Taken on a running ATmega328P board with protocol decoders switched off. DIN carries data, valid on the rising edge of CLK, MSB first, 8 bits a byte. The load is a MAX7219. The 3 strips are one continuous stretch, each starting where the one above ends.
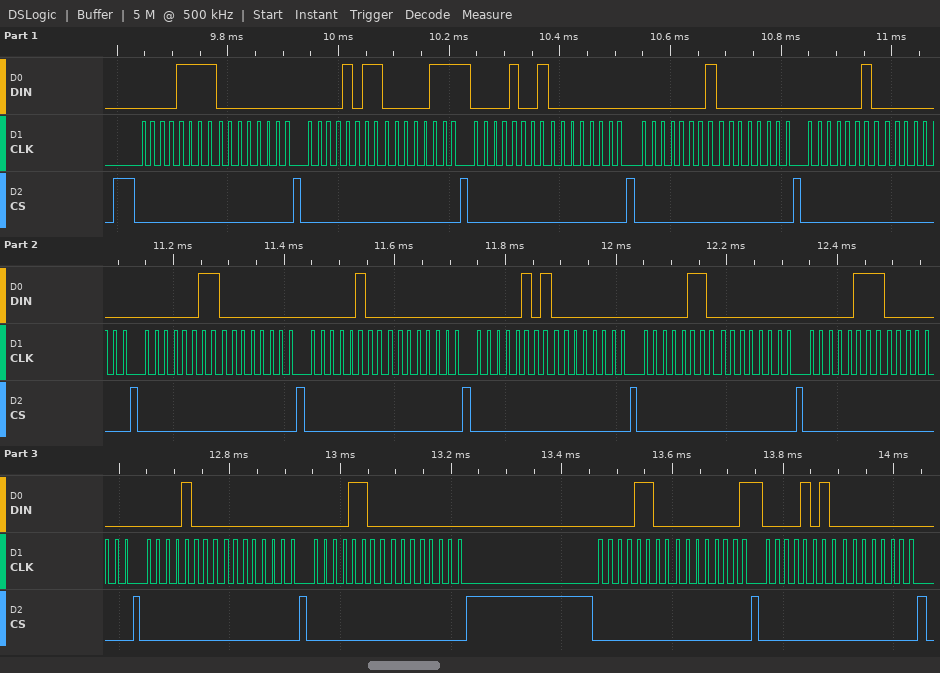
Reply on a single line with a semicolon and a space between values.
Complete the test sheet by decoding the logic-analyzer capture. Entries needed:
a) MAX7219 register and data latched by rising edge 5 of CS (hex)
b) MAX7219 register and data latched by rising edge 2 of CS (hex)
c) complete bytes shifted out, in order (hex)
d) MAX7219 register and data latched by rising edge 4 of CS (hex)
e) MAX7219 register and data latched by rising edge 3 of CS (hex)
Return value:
register 0x1, data 0x00; register 0xF, data 0x00; 0F 00 0B 07 09 00 01 00 02 00 03 00 04 00 05 00 06 00 07 00 08 00 0C 00 0C 01 0A 00; register 0x9, data 0x00; register 0xB, data 0x07
